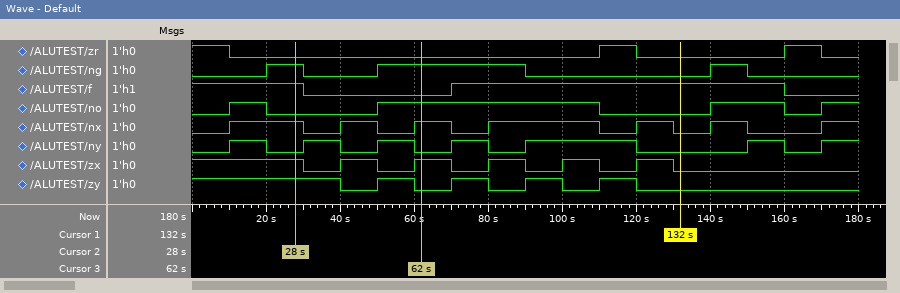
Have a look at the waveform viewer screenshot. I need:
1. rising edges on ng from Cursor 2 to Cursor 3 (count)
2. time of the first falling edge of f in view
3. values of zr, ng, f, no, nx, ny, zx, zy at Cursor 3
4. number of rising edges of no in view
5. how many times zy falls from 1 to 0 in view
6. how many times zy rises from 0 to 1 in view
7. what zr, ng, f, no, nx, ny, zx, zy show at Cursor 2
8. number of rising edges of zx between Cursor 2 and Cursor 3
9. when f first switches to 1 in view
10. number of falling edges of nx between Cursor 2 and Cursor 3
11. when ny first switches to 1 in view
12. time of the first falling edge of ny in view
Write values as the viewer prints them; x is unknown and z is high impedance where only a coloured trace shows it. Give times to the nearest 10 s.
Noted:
1
30 s
zr=0, ng=1, f=0, no=1, nx=1, ny=0, zx=1, zy=0
4
5
4
zr=0, ng=1, f=1, no=0, nx=1, ny=0, zx=1, zy=1
2
70 s
2
10 s
20 s
